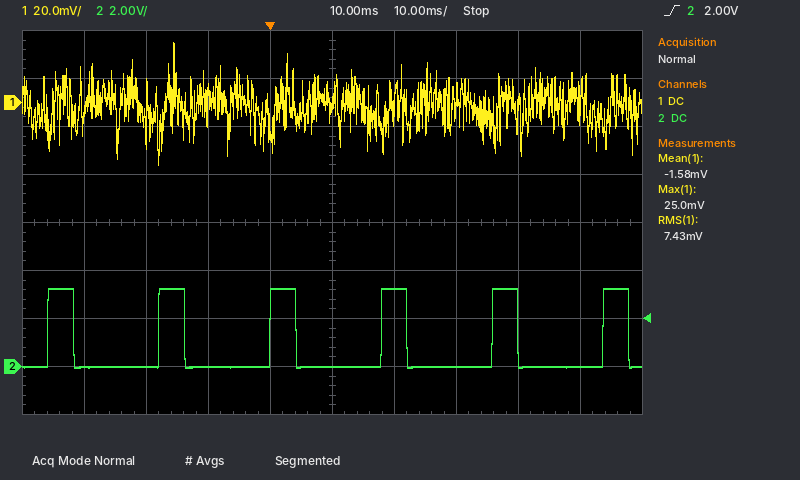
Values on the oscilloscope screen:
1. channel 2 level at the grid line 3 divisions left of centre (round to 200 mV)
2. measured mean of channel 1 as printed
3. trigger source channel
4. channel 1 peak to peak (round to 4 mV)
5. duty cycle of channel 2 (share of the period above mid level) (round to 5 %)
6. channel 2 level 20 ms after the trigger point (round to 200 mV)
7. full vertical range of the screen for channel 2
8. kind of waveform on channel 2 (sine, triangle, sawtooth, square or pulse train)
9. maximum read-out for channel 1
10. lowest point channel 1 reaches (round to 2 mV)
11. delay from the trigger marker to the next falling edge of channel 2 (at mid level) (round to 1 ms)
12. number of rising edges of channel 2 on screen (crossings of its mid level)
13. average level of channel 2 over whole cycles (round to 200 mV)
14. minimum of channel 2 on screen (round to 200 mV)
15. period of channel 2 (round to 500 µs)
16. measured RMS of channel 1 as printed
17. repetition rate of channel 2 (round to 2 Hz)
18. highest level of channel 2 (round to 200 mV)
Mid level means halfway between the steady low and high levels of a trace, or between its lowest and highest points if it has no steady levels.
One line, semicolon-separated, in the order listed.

0.0 V; -1.58 mV; channel 2; 52 mV; 25 %; 3.2 V; 16 V; pulse train; 25.0 mV; -26 mV; 4 ms; 6; 800 mV; 0.0 V; 18.0 ms; 7.43 mV; 56 Hz; 3.2 V
